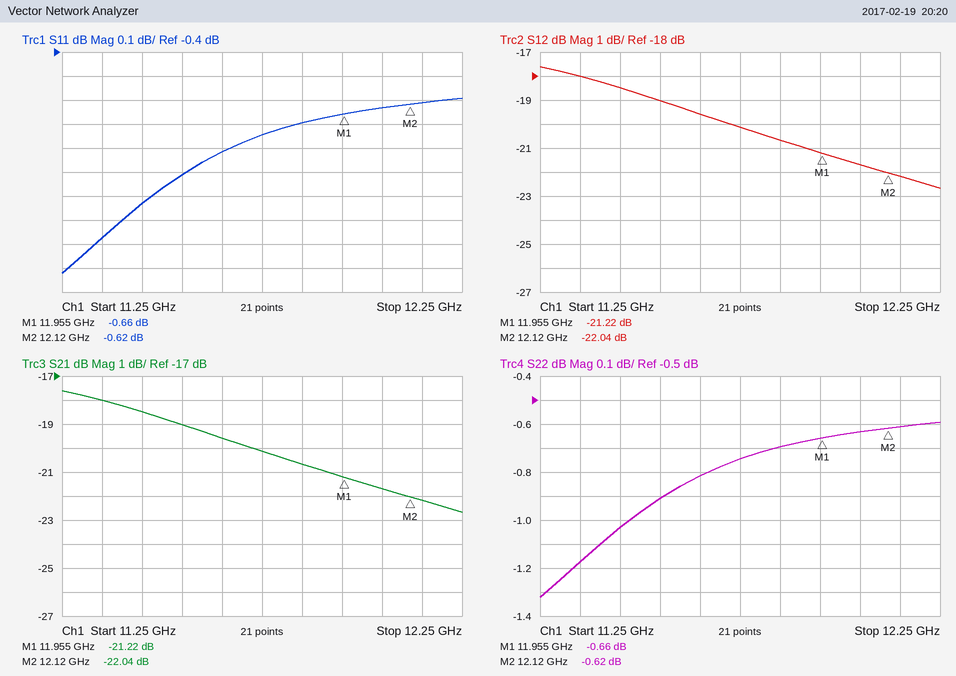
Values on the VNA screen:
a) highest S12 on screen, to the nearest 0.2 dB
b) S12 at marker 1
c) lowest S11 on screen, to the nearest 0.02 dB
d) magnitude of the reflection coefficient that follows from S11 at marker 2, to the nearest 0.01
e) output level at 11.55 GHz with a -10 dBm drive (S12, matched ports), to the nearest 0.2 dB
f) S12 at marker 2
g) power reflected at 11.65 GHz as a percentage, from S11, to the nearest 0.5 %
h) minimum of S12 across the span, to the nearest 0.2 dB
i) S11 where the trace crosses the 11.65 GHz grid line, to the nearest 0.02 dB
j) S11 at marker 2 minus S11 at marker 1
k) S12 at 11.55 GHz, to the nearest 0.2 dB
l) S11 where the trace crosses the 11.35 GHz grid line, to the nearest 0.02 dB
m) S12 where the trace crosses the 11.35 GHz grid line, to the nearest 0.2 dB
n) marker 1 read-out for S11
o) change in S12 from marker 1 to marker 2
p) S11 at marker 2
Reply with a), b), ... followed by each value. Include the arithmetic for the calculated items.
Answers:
a) -17.6 dB
b) -21.22 dB
c) -1.32 dB
d) 10^(-0.62/20) ≈ 0.93
e) -10 dBm + (-19.0 dB) = -29.0 dBm
f) -22.04 dB
g) 10^(-0.82/10) ≈ 82.8 %, so 83.0 % to the nearest 0.5 %
h) -22.6 dB
i) -0.82 dB
j) -0.62 − (-0.66) = 0.04 dB
k) -19.0 dB
l) -1.18 dB
m) -18.0 dB
n) -0.66 dB
o) -22.04 − (-21.22) = -0.82 dB
p) -0.62 dB
